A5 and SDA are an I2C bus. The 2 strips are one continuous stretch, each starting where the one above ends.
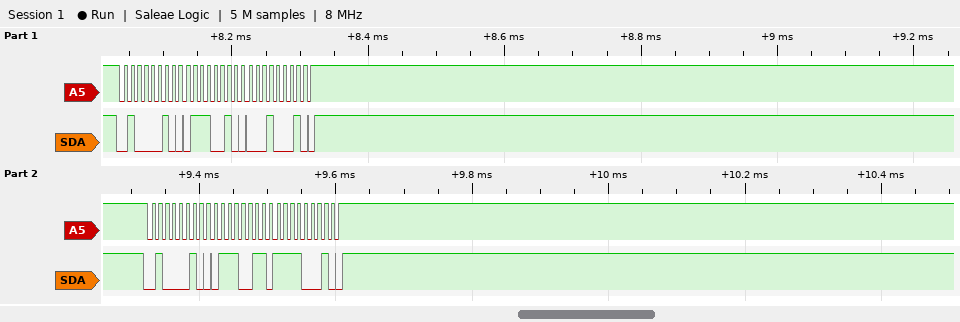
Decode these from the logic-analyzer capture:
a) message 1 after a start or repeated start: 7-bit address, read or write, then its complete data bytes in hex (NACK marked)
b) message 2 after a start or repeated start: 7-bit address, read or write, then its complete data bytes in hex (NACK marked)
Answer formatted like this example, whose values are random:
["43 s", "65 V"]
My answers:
["0x21 write: 72 11", "0x21 write: 73 F1"]
